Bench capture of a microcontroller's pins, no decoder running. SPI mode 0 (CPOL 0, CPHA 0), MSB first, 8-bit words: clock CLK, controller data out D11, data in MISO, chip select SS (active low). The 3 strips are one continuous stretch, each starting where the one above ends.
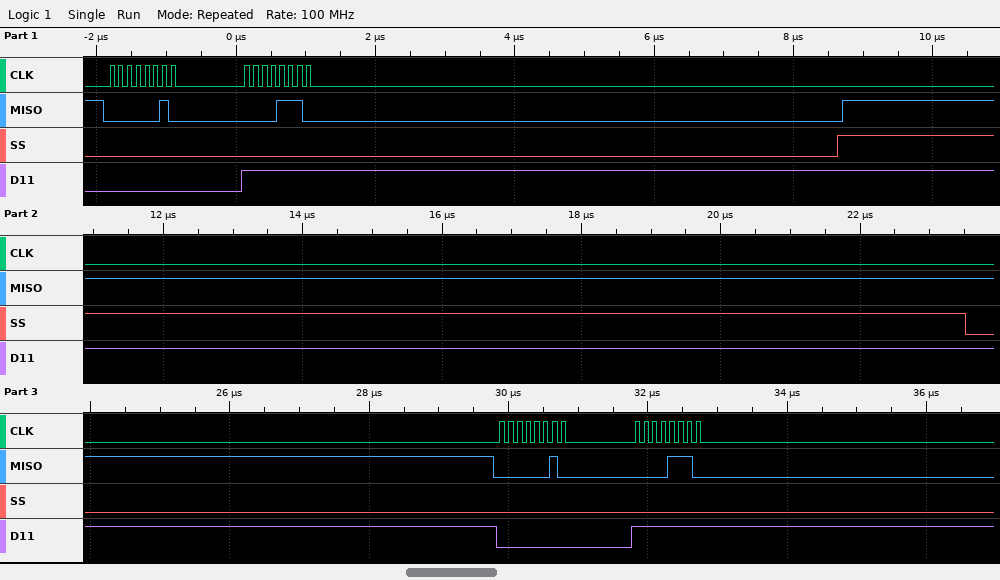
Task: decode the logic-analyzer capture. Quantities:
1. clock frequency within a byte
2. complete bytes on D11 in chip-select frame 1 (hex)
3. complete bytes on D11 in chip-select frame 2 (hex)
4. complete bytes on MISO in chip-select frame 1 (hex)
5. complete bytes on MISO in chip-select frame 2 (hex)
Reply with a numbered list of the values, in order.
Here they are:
1. 8 MHz
2. 00 FF
3. 00 FF
4. 02 0E
5. 02 0E
